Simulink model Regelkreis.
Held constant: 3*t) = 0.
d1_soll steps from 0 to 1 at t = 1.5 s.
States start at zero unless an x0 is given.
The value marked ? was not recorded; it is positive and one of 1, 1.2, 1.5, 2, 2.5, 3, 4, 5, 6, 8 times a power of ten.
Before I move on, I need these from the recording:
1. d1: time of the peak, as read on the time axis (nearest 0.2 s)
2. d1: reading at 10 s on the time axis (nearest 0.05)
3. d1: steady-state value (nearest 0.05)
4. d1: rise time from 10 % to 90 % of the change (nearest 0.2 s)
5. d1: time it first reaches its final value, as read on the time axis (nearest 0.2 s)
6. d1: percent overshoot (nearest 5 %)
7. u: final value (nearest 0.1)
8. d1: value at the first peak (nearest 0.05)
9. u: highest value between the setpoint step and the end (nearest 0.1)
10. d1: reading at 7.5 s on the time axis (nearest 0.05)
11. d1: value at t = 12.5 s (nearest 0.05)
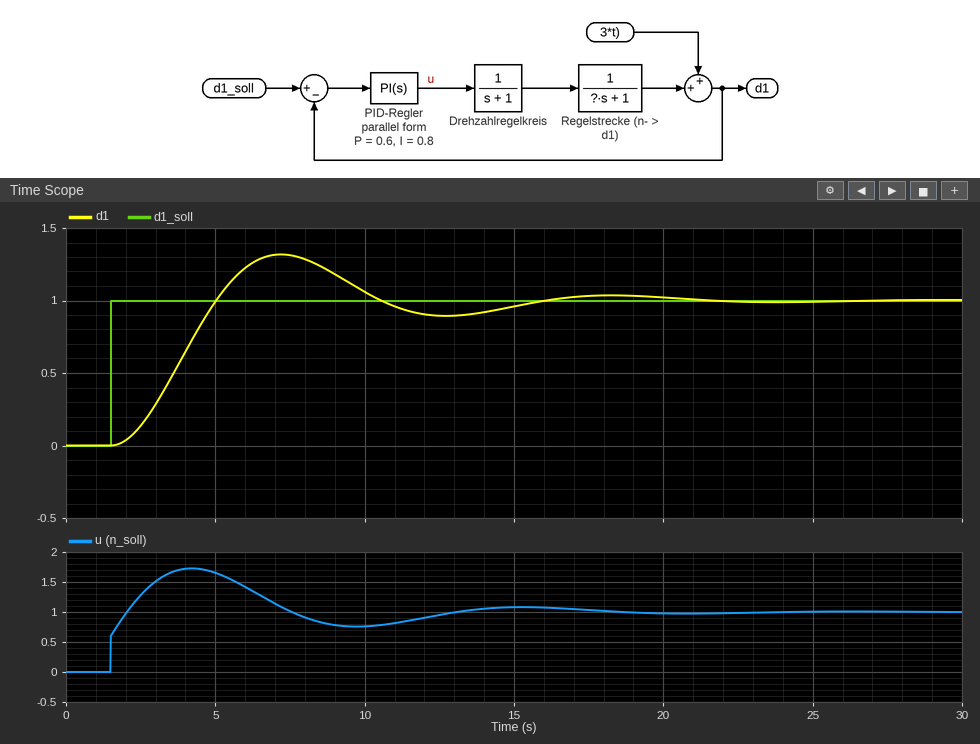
7.2 s
1.05
1.00
2.4 s
5.0 s
30 %
1.0
1.30
1.7
1.30
0.90
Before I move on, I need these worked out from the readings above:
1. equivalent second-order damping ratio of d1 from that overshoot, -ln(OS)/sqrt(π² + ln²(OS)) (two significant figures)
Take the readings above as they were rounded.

0.36
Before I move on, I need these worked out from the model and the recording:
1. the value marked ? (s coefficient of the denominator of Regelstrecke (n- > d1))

2
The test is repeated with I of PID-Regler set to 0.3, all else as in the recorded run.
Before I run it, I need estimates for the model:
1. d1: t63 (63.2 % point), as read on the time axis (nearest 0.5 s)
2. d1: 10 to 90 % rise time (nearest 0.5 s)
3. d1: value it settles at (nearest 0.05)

5.0 s
5.5 s
1.00
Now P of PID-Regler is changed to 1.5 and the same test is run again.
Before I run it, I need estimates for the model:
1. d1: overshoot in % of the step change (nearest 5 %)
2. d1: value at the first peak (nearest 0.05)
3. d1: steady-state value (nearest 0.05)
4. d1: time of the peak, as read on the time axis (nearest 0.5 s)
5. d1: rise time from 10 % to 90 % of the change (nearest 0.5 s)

15 %
1.15
1.00
6.0 s
2.0 s
